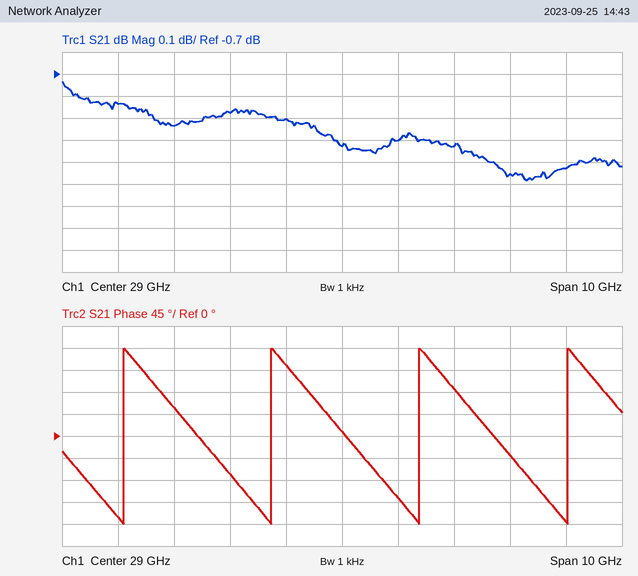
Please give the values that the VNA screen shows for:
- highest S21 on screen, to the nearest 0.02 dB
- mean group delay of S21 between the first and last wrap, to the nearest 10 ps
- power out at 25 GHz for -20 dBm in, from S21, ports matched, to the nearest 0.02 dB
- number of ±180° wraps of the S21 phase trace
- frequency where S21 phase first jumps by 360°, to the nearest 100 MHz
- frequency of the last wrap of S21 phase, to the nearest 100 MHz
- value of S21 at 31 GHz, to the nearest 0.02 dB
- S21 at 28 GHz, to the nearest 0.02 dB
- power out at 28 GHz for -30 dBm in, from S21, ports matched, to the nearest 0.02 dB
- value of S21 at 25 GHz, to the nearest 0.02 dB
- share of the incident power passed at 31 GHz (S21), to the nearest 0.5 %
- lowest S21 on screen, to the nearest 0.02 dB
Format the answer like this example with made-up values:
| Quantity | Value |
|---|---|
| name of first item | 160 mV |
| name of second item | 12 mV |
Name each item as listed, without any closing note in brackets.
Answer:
| Quantity | Value |
|---|---|
| highest S21 on screen, to the nearest 0.02 dB | -0.74 dB |
| mean group delay of S21 between the first and last wrap, to the nearest 10 ps | 380 ps |
| power out at 25 GHz for -20 dBm in, from S21, ports matched, to the nearest 0.02 dB | -20.84 dBm |
| number of ±180° wraps of the S21 phase trace | 4 |
| frequency where S21 phase first jumps by 360°, to the nearest 100 MHz | 25.1 GHz |
| frequency of the last wrap of S21 phase, to the nearest 100 MHz | 33.0 GHz |
| value of S21 at 31 GHz, to the nearest 0.02 dB | -1.02 dB |
| S21 at 28 GHz, to the nearest 0.02 dB | -0.90 dB |
| power out at 28 GHz for -30 dBm in, from S21, ports matched, to the nearest 0.02 dB | -30.90 dBm |
| value of S21 at 25 GHz, to the nearest 0.02 dB | -0.84 dB |
| share of the incident power passed at 31 GHz (S21), to the nearest 0.5 % | 79.0 % |
| lowest S21 on screen, to the nearest 0.02 dB | -1.18 dB |
